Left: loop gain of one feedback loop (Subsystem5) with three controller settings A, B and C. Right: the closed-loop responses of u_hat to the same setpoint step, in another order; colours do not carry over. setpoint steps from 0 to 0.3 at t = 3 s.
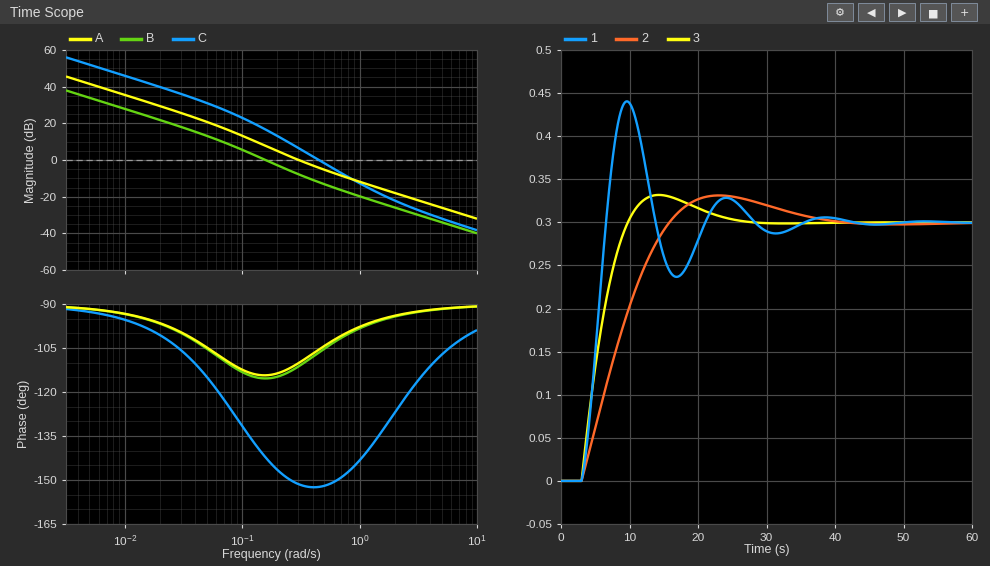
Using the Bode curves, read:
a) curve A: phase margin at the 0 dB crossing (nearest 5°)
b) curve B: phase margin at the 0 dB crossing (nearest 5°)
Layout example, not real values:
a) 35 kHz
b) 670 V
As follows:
a) 70°
b) 65°
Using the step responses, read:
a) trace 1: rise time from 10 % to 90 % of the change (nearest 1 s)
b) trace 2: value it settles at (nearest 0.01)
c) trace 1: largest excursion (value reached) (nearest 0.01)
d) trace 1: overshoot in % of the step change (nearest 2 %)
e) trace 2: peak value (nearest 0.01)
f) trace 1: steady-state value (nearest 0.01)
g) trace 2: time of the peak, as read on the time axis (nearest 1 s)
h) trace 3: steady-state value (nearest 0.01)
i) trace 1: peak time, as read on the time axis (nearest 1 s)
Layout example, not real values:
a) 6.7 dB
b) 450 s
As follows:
a) 3 s
b) 0.30
c) 0.44
d) 46 %
e) 0.33
f) 0.30
g) 23 s
h) 0.30
i) 10 s
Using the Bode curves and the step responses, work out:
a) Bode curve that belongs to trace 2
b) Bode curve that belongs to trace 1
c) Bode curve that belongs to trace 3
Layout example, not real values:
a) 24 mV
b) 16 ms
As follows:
a) B
b) C
c) A
